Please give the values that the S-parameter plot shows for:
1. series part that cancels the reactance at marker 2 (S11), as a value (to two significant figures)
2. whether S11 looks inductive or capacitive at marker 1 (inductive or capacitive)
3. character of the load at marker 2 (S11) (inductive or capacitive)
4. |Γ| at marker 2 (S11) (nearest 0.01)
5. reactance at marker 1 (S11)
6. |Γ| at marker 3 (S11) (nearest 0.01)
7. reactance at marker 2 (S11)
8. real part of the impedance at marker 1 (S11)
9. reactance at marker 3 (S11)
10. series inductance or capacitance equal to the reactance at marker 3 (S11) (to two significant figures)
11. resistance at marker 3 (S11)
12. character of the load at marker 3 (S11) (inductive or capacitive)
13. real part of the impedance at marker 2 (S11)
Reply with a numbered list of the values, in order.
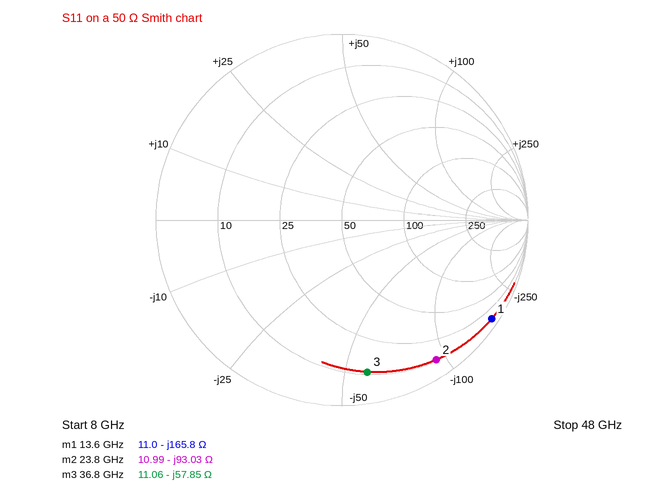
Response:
1. 620 pH
2. capacitive
3. capacitive
4. 0.91
5. -165.8 Ω
6. 0.83
7. -93.03 Ω
8. 11.0 Ω
9. -57.85 Ω
10. 75 fF
11. 11.06 Ω
12. capacitive
13. 10.99 Ω
